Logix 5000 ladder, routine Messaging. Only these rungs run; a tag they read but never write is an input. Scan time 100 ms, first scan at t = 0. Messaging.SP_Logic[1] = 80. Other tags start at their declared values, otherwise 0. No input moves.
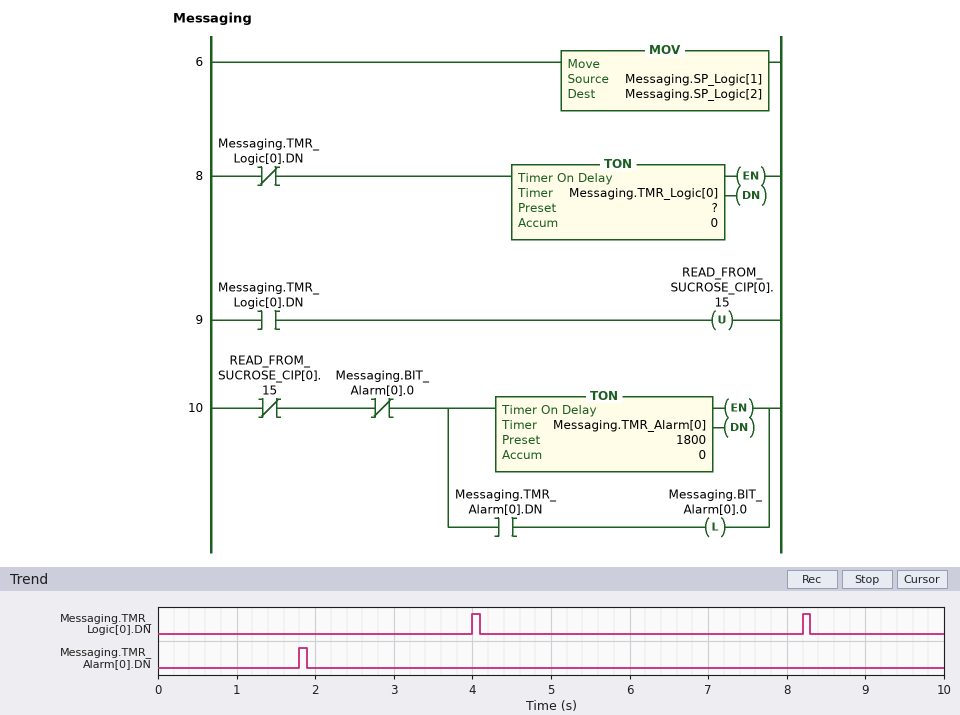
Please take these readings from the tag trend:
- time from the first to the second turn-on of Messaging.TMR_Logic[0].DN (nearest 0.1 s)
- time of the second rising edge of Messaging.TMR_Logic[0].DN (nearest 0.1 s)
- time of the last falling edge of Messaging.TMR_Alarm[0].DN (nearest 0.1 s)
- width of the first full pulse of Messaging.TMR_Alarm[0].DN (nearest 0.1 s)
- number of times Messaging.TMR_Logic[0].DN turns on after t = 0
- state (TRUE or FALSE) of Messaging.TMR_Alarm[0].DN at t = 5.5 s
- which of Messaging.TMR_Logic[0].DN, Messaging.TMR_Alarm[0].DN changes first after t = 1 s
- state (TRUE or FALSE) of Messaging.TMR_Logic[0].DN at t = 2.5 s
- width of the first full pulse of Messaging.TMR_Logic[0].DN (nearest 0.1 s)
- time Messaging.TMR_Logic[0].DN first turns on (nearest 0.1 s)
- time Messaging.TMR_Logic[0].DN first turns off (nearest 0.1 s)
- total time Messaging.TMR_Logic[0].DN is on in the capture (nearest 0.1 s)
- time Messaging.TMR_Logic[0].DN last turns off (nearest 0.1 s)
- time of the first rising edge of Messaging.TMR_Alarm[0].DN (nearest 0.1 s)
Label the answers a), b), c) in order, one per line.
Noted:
a) 4.2 s
b) 8.2 s
c) 1.9 s
d) 0.1 s
e) 2
f) FALSE
g) Messaging.TMR_Alarm[0].DN
h) FALSE
i) 0.1 s
j) 4.0 s
k) 4.1 s
l) 0.2 s
m) 8.3 s
n) 1.8 s
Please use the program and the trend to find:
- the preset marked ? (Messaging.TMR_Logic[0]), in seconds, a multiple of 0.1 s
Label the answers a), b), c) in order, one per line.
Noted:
a) 4.0 s
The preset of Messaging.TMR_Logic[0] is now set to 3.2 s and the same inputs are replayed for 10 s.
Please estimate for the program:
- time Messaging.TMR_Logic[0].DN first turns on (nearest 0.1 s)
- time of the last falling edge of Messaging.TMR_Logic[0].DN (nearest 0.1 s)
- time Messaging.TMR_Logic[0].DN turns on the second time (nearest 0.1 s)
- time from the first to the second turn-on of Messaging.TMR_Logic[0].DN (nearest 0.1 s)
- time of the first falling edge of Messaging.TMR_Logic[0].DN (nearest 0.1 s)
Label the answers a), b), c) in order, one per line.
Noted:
a) 3.2 s
b) 6.7 s
c) 6.6 s
d) 3.4 s
e) 3.3 s
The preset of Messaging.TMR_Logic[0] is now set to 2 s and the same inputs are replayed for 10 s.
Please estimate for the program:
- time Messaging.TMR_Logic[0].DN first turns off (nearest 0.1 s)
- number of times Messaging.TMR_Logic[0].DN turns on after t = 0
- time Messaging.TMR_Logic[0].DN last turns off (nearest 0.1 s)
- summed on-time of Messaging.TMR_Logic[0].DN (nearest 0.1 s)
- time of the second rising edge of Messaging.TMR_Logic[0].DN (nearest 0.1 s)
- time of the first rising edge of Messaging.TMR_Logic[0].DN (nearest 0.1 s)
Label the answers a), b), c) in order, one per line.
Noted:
a) 2.1 s
b) 4
c) 8.7 s
d) 0.4 s
e) 4.2 s
f) 2.0 s
